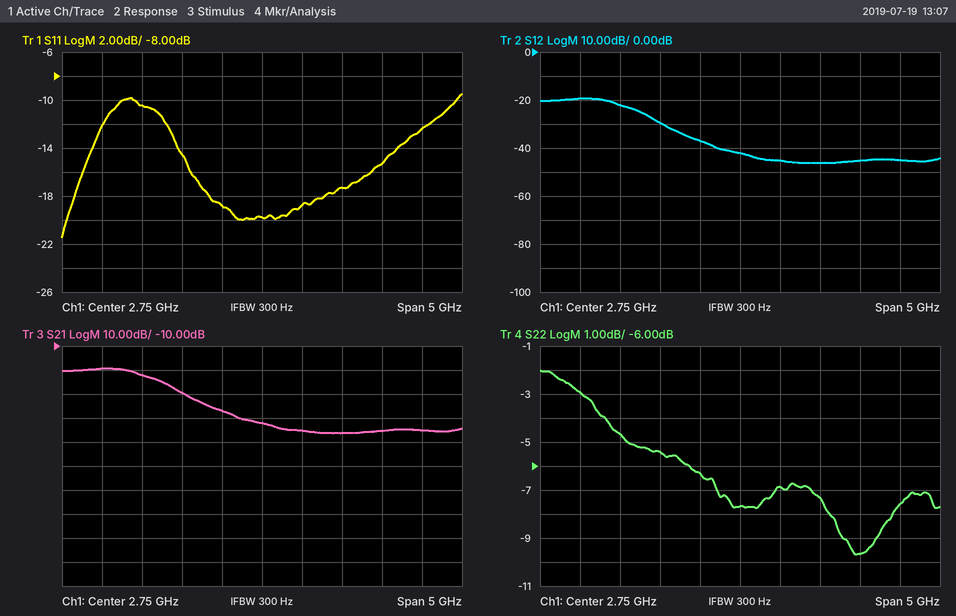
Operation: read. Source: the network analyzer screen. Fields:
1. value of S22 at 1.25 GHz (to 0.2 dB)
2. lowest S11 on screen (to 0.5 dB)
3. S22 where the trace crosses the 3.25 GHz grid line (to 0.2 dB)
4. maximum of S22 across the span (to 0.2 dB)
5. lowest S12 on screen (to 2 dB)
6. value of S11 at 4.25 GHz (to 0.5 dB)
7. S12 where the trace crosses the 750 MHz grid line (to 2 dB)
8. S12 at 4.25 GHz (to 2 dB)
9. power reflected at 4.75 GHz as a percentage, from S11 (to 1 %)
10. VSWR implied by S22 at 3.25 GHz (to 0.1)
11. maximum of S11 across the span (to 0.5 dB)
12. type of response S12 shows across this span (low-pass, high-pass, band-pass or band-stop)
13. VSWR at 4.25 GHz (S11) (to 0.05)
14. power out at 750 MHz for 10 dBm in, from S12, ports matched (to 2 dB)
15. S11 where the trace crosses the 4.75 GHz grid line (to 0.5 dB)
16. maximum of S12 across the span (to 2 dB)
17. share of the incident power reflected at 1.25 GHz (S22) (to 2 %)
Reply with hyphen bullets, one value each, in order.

- -4.6 dB
- -21.5 dB
- -6.8 dB
- -2.0 dB
- -46 dB
- -15.5 dB
- -20 dB
- -46 dB
- 6 %
- 2.7
- -9.5 dB
- low-pass
- 1.40
- -10 dBm
- -12.5 dB
- -20 dB
- 34 %
